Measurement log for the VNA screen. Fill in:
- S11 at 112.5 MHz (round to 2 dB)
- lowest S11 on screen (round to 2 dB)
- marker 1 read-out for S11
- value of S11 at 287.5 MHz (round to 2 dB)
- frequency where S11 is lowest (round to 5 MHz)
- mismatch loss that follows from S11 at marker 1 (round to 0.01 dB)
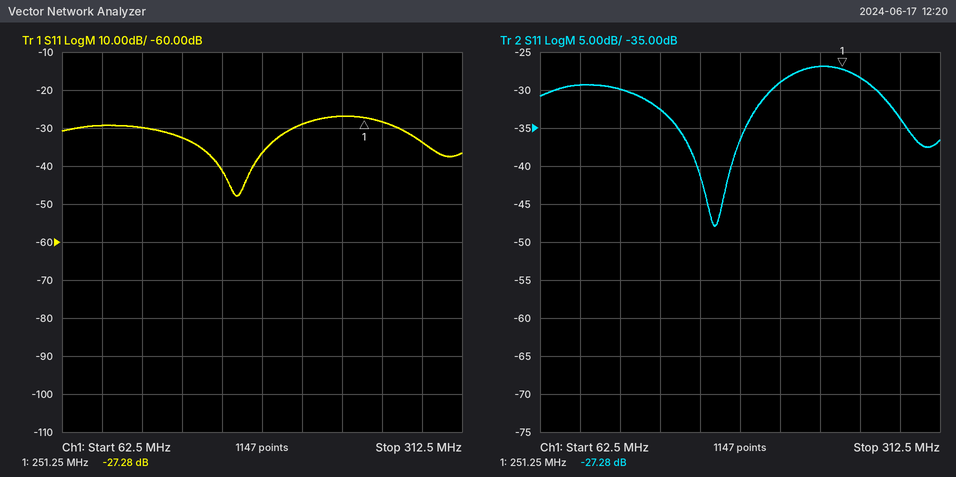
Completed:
-30 dB
-48 dB
-27.28 dB
-34 dB
170 MHz
0.01 dB
